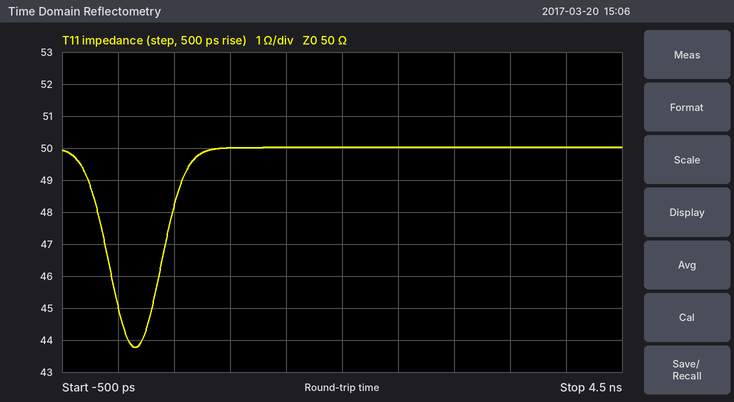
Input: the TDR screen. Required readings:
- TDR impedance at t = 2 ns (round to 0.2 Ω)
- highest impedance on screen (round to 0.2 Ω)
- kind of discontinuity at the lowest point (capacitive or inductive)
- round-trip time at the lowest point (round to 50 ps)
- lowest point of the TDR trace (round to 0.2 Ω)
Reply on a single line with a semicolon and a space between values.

50.0 Ω; 50.0 Ω; capacitive; 150 ps; 43.8 Ω
